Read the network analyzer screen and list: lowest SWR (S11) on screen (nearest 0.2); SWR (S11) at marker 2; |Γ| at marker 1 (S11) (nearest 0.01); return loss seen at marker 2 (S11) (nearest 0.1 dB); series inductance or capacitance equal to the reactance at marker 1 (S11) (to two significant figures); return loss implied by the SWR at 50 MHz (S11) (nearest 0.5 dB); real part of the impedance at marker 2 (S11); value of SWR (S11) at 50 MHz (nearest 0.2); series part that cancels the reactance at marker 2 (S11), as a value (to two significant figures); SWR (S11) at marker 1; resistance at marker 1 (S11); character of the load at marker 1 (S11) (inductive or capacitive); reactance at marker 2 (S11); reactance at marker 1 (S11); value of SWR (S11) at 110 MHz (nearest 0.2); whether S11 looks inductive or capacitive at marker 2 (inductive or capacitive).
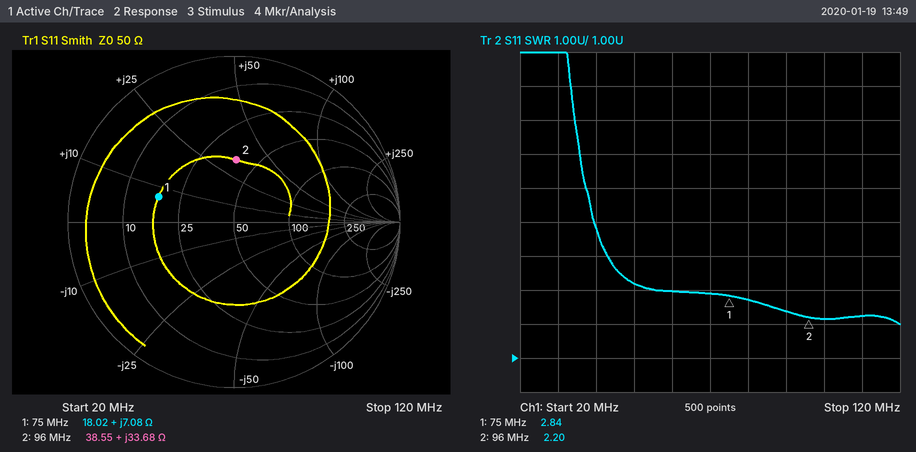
2.0
2.20
0.48
8.5 dB
15 nH
5.5 dB
38.55 Ω
3.2
49 pF
2.84
18.02 Ω
inductive
+33.68 Ω
+7.08 Ω
2.2
inductive
